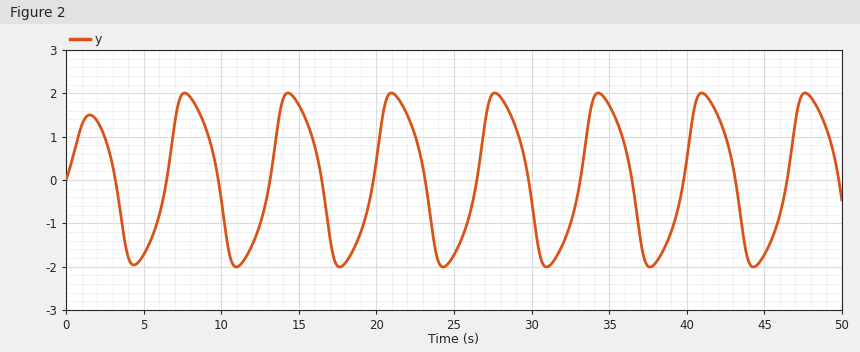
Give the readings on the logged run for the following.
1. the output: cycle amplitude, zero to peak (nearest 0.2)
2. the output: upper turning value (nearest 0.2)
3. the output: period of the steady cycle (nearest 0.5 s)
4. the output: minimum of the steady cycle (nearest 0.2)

2.0
2.0
6.5 s
-2.0
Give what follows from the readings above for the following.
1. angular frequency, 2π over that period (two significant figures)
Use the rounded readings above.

0.97 rad/s
